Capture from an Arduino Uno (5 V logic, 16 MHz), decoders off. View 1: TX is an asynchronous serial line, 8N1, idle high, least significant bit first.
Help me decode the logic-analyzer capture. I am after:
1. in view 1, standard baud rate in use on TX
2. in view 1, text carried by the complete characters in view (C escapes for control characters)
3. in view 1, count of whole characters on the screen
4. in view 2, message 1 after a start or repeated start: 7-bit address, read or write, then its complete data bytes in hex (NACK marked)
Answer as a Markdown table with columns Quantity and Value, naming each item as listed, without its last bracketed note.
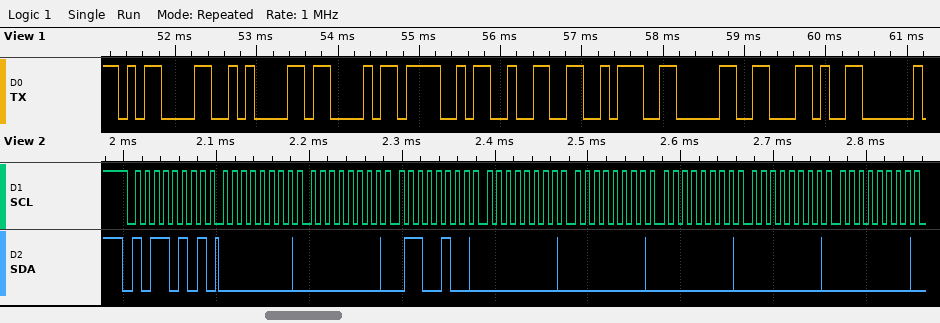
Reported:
| Quantity | Value |
|---|---|
| in view 1, standard baud rate in use on TX | 9600 baud |
| in view 1, text carried by the complete characters in view | "\r\nCO2:0," |
| in view 1, count of whole characters on the screen | 8 |
| in view 2, message 1 after a start or repeated start: 7-bit address, read or write, then its complete data bytes in hex | 0x5A read: 00 00 64 00 00 00 00 00 |
